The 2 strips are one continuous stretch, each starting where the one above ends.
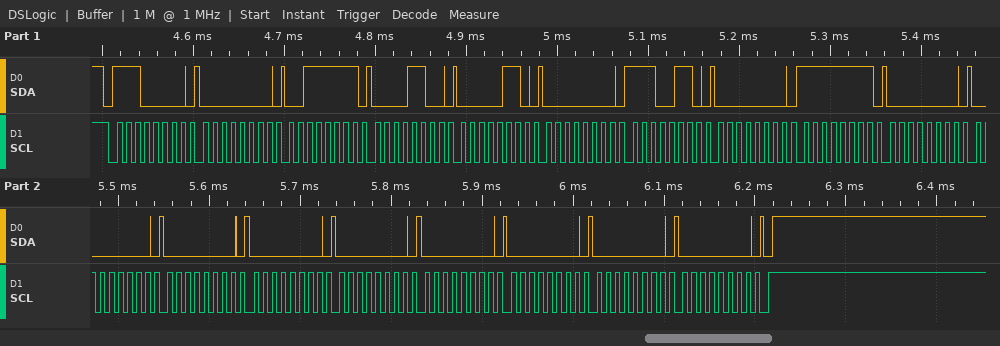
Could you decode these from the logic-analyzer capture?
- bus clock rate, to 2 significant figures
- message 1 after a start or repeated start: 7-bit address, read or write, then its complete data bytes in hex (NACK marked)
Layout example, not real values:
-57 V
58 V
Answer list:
100 kHz
0x70 write: 00 3F 0C 06 00 E6 00 FF 00 00 00 00 00 00 00 00 00
